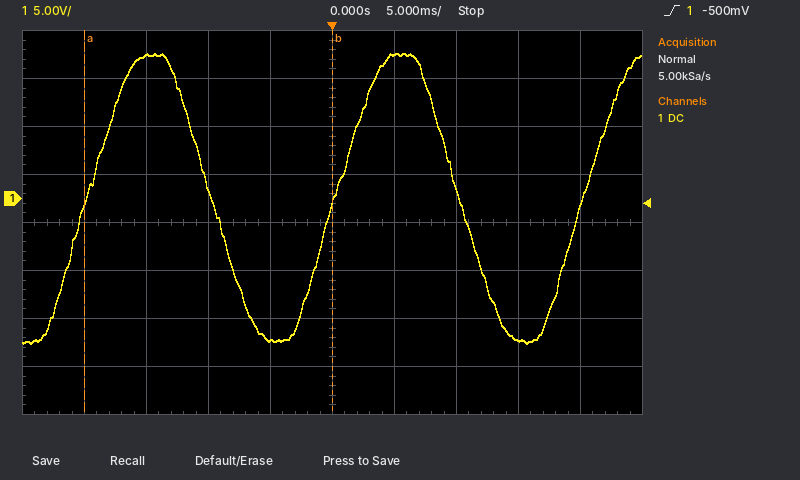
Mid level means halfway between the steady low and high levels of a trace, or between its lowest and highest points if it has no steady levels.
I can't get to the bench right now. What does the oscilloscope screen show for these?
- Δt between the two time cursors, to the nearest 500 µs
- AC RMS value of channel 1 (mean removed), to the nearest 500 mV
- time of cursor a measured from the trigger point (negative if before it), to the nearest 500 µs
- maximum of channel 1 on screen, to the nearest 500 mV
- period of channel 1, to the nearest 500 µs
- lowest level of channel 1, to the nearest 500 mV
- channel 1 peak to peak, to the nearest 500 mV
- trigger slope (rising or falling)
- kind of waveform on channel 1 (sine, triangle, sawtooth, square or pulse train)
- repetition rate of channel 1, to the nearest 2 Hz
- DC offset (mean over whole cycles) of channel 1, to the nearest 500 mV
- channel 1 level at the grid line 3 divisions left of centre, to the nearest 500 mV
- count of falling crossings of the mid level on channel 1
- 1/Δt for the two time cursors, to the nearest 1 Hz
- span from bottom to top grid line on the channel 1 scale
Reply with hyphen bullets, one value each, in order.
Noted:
- 20.0 ms
- 10.5 V
- -20.0 ms
- 15.0 V
- 20.0 ms
- -15.0 V
- 30.0 V
- rising
- sine
- 50 Hz
- 0.0 V
- 15.0 V
- 2
- 50 Hz
- 40 V
